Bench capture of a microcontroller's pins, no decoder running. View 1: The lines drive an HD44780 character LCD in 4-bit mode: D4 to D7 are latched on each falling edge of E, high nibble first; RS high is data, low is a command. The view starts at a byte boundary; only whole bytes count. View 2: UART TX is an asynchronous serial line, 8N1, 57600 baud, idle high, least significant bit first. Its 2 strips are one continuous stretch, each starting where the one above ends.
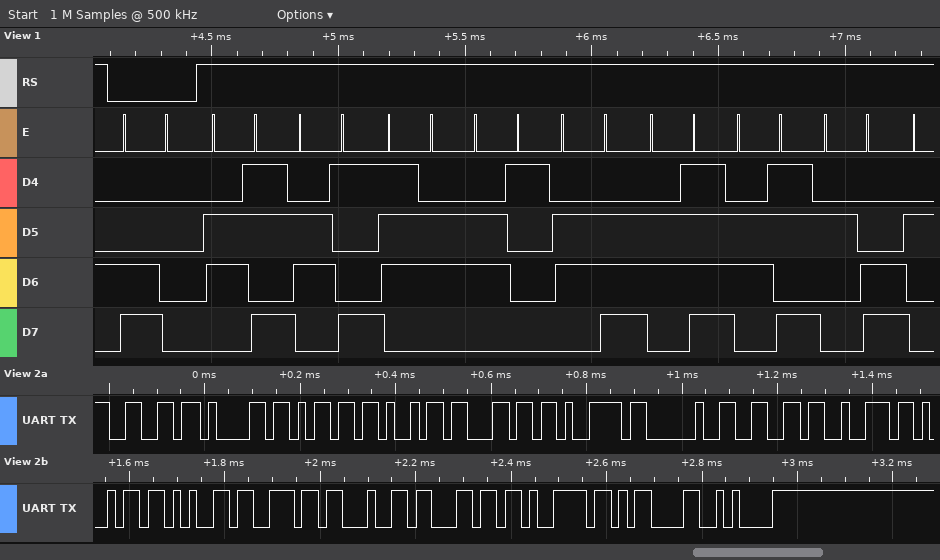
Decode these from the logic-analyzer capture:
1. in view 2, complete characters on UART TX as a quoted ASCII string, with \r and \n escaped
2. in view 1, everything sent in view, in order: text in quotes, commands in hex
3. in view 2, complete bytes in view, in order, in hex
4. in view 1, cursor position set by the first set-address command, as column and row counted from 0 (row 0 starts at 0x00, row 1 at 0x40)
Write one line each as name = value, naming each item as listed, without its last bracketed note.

in view 2, complete characters on UART TX as a quoted ASCII string, with \r and \n escaped = "family friendly\r\n"
in view 1, everything sent in view, in order: text in quotes, commands in hex = 0xC0 "kivanok,"
in view 2, complete bytes in view, in order, in hex = 66 61 6D 69 6C 79 20 66 72 69 65 6E 64 6C 79 0D 0A
in view 1, cursor position set by the first set-address command, as column and row counted from 0 = column 0, row 1
